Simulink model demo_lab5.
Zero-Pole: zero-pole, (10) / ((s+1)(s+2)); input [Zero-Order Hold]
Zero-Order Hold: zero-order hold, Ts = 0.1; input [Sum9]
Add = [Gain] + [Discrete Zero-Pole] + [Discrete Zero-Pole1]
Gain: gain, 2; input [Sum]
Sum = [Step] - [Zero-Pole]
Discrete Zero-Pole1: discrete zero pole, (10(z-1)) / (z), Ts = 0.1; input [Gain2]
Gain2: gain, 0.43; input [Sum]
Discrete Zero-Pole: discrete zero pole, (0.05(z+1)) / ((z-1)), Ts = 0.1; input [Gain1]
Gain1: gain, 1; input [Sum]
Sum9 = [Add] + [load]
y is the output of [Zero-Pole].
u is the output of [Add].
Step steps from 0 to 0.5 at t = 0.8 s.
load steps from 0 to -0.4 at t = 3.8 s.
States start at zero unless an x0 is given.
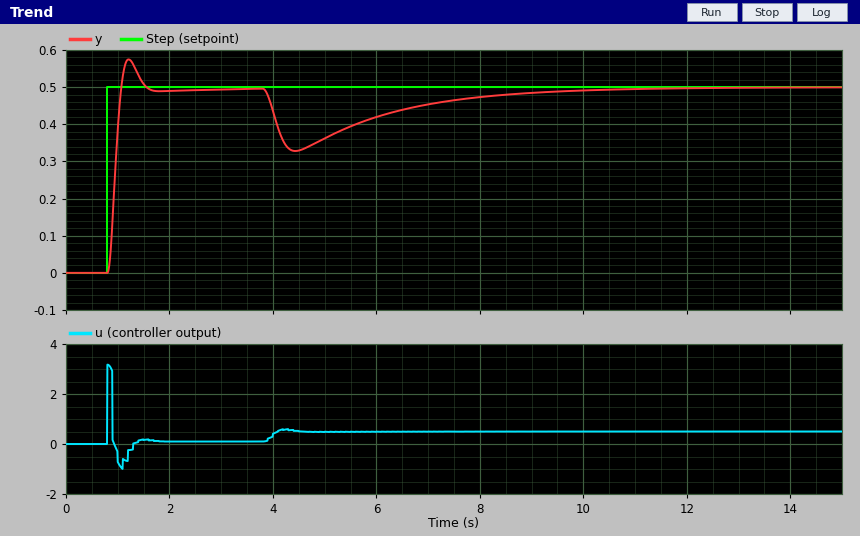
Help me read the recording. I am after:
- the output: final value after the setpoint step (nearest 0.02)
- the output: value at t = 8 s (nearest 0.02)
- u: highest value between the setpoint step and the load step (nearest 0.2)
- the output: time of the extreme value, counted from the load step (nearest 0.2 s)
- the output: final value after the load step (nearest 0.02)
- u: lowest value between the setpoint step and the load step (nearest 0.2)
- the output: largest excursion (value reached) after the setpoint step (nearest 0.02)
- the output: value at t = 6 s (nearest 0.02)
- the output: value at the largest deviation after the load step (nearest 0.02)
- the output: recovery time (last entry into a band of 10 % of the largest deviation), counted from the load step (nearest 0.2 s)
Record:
0.50
0.48
3.2
0.6 s
0.50
-1.0
0.58
0.42
0.32
5.0 s
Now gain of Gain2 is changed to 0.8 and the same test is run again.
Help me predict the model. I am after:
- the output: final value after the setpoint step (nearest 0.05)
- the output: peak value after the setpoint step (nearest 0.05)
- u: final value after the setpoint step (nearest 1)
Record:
0.50
0.60
0
